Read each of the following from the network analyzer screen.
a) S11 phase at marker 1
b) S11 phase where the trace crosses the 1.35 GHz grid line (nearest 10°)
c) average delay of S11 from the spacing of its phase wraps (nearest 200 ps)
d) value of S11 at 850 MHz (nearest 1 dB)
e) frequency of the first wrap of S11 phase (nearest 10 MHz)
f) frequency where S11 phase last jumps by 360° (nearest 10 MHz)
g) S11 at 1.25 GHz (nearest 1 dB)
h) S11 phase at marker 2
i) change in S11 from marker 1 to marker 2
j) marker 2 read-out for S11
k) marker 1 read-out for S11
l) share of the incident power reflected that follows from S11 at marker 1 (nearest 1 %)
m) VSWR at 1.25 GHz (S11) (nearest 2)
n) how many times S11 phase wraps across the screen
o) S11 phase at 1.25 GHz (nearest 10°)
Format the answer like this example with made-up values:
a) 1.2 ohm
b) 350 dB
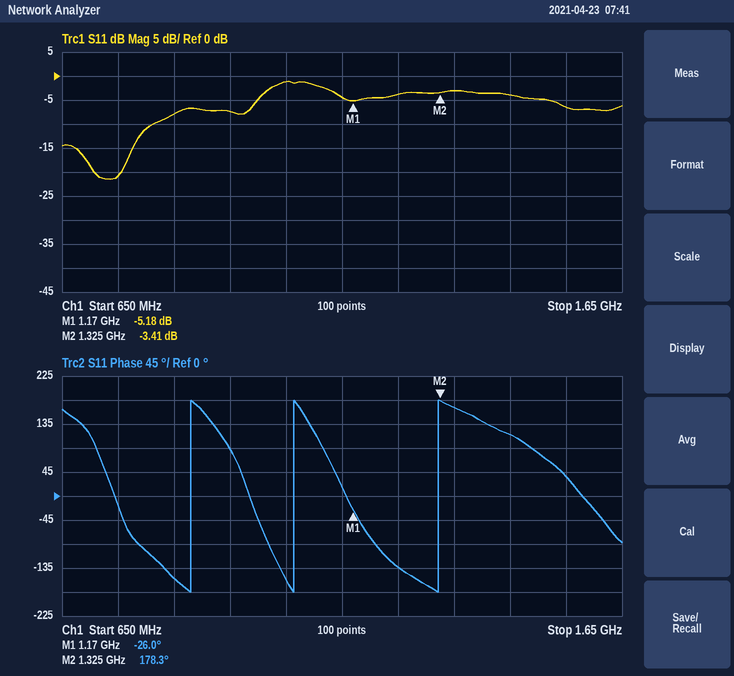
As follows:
a) -26.0°
b) 170°
c) 4.6 ns
d) -8 dB
e) 880 MHz
f) 1.32 GHz
g) -4 dB
h) 178.3°
i) 1.77 dB
j) -3.41 dB
k) -5.18 dB
l) 30 %
m) 4
n) 3
o) -130°
